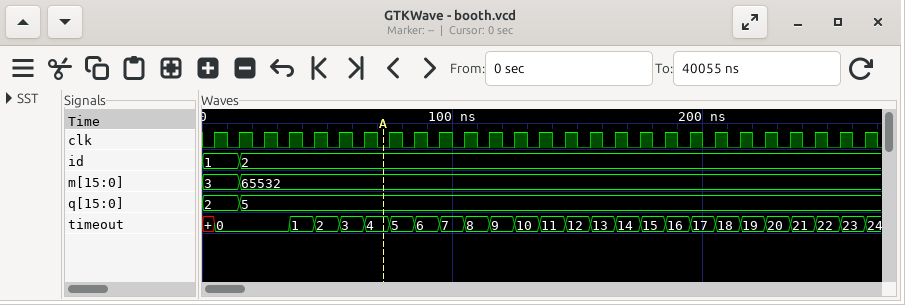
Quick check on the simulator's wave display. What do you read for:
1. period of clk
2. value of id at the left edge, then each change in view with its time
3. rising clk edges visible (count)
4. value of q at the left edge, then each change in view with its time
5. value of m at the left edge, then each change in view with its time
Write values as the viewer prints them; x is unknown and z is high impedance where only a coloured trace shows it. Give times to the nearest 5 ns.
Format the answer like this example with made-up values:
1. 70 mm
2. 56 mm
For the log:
1. 10 ns
2. 1, 2 at 15 ns
3. 27
4. 2, 5 at 15 ns
5. 3, 65532 at 15 ns
